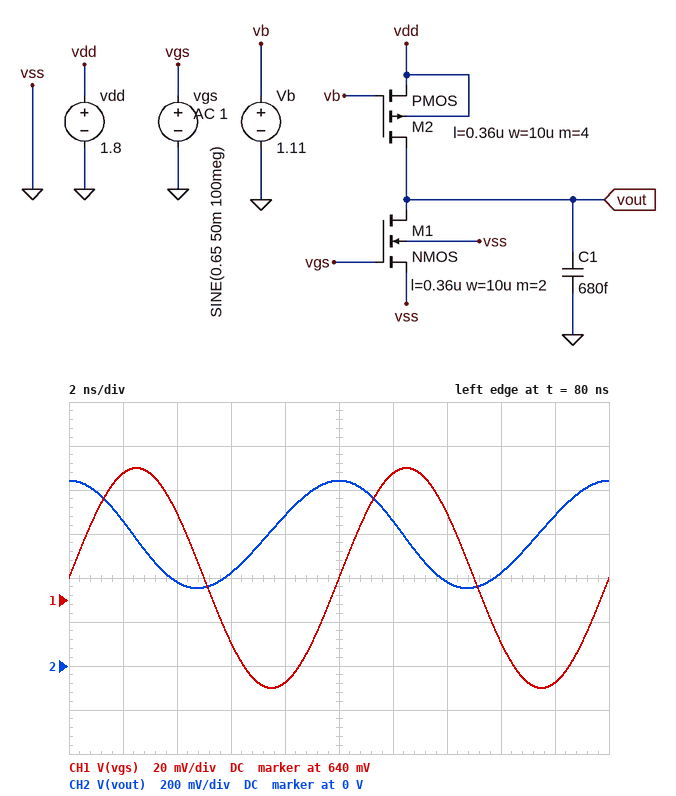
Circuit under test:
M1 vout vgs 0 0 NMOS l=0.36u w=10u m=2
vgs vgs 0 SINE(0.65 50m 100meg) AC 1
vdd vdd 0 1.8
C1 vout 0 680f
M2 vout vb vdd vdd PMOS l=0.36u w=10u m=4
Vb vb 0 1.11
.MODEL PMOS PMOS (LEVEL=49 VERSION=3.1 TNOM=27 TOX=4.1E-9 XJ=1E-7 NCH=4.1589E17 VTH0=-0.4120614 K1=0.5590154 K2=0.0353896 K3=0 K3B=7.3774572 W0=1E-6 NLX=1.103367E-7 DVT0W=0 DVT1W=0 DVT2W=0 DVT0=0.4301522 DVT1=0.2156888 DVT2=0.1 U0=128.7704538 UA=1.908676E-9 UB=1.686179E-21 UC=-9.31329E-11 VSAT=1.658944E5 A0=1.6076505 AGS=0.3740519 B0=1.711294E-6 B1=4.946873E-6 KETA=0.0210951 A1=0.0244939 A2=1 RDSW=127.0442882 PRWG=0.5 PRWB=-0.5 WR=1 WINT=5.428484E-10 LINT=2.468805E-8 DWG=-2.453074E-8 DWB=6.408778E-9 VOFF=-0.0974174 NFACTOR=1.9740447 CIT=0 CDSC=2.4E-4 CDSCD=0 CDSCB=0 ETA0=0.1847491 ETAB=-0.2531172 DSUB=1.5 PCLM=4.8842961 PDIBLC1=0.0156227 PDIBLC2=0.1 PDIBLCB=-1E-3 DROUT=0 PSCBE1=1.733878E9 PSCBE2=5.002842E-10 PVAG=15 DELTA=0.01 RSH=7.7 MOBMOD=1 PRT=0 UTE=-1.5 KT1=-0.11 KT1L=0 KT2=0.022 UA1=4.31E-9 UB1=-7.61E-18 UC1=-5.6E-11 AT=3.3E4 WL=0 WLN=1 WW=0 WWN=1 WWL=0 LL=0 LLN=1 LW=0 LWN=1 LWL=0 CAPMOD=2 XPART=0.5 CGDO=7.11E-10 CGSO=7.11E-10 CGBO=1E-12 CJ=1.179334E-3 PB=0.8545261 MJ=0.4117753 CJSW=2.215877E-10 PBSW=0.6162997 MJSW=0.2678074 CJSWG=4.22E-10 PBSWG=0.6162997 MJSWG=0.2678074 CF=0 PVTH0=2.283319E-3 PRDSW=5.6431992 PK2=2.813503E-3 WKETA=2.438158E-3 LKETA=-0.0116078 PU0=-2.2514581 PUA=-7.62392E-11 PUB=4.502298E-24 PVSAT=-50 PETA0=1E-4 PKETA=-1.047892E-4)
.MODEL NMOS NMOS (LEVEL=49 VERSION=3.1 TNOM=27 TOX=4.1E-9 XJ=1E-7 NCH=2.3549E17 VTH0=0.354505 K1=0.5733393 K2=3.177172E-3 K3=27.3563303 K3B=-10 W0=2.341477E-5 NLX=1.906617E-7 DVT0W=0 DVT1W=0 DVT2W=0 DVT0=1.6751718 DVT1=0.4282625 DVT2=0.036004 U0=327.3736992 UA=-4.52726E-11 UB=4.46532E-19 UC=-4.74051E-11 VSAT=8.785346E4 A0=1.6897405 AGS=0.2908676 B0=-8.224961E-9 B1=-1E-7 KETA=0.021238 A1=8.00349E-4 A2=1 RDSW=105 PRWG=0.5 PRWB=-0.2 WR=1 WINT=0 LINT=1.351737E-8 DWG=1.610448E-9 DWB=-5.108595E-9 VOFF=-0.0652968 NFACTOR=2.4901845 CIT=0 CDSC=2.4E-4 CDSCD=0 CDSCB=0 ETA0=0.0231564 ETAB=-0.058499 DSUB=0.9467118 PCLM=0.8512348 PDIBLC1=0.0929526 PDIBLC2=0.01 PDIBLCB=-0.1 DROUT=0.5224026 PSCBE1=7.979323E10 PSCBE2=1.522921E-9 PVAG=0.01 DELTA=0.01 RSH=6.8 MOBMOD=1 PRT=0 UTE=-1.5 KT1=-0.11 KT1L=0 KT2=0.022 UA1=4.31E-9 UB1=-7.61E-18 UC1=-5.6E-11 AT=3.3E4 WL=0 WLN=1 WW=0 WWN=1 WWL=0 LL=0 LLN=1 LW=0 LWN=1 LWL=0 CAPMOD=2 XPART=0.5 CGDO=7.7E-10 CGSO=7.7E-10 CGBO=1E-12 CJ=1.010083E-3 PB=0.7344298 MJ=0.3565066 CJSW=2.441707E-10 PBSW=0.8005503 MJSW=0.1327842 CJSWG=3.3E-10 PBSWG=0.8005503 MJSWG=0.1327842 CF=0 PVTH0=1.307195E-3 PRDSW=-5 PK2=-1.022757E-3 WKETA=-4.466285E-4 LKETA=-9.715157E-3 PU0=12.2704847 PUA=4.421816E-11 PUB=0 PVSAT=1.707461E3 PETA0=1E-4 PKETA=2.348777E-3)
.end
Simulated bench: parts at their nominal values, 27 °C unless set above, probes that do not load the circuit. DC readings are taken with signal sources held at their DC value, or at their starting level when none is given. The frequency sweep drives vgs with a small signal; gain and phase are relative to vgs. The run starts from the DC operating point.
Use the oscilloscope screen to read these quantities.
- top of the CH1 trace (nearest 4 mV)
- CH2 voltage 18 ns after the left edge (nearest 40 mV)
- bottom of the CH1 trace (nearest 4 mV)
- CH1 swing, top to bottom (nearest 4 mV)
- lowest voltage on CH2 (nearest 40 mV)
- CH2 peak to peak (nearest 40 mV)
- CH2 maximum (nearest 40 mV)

700 mV
680 mV
600 mV
100 mV
360 mV
480 mV
840 mV
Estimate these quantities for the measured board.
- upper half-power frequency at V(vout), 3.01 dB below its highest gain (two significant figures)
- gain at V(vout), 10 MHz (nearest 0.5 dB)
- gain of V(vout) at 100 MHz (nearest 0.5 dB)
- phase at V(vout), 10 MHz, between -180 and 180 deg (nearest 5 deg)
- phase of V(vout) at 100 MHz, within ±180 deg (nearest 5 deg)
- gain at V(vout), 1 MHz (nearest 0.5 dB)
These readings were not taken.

8.2 MHz
32.0 dB
14.0 dB
130 deg
95 deg
35.5 dB
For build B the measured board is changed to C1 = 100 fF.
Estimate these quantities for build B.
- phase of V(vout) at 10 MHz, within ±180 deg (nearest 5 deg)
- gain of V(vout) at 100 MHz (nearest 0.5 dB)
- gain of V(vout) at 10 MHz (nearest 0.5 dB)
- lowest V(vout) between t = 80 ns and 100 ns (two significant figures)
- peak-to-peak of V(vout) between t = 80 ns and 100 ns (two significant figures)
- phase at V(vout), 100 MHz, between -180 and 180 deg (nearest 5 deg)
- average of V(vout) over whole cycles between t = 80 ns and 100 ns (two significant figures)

165 deg
26.5 dB
35.5 dB
93 mV
1.6 V
110 deg
850 mV
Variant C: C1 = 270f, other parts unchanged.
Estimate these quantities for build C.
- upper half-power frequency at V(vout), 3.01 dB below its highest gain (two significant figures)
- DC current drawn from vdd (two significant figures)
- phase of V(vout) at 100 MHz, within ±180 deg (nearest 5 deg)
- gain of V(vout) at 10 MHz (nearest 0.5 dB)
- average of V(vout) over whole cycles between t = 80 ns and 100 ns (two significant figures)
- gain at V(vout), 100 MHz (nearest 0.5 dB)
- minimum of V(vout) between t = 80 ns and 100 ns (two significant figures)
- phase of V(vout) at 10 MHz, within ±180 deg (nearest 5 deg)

18 MHz
190 µA
100 deg
34.5 dB
670 mV
21.0 dB
150 mV
150 deg
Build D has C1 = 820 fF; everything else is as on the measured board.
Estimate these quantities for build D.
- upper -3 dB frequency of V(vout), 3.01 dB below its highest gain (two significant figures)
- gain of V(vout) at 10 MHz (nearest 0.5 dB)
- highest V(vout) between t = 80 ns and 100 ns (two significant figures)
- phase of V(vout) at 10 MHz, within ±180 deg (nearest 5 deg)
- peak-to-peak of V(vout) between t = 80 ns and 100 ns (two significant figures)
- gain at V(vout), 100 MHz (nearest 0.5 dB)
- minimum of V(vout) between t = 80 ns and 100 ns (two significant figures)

6.9 MHz
31.0 dB
800 mV
125 deg
410 mV
12.5 dB
390 mV
